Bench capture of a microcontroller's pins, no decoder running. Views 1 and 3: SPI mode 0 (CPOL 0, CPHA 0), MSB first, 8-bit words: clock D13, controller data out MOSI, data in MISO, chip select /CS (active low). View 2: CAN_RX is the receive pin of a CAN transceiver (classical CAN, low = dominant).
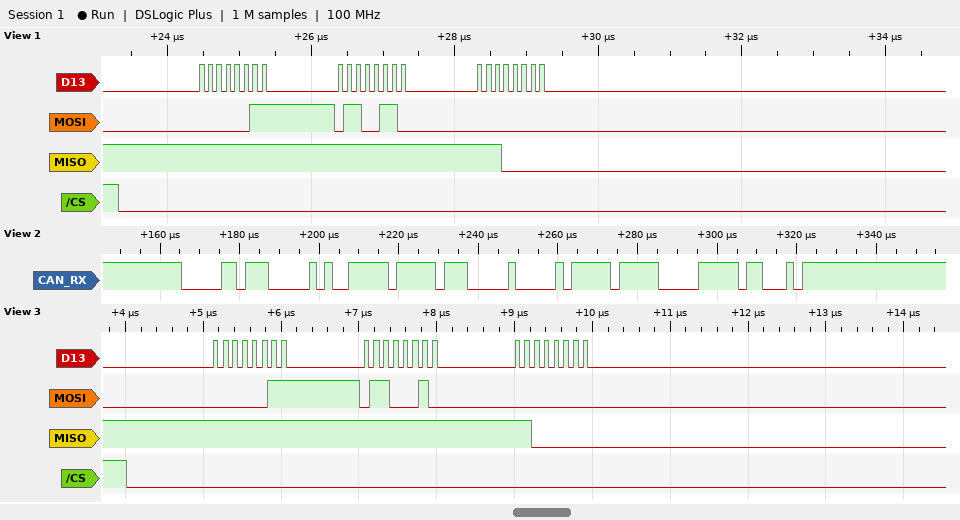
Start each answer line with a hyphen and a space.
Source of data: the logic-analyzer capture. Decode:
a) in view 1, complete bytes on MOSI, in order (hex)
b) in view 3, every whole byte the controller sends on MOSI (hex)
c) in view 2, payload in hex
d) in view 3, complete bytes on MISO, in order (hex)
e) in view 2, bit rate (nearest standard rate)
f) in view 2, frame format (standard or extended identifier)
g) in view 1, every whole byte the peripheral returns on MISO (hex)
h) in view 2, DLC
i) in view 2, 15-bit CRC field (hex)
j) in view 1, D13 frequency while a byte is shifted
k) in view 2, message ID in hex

- 03 66 00
- 03 62 00
- FF F8 00 FF
- FF FF C0
- 500 kbit/s
- standard
- FF FF E0
- 4
- 0x61F8
- 8 MHz
- 0x05C
